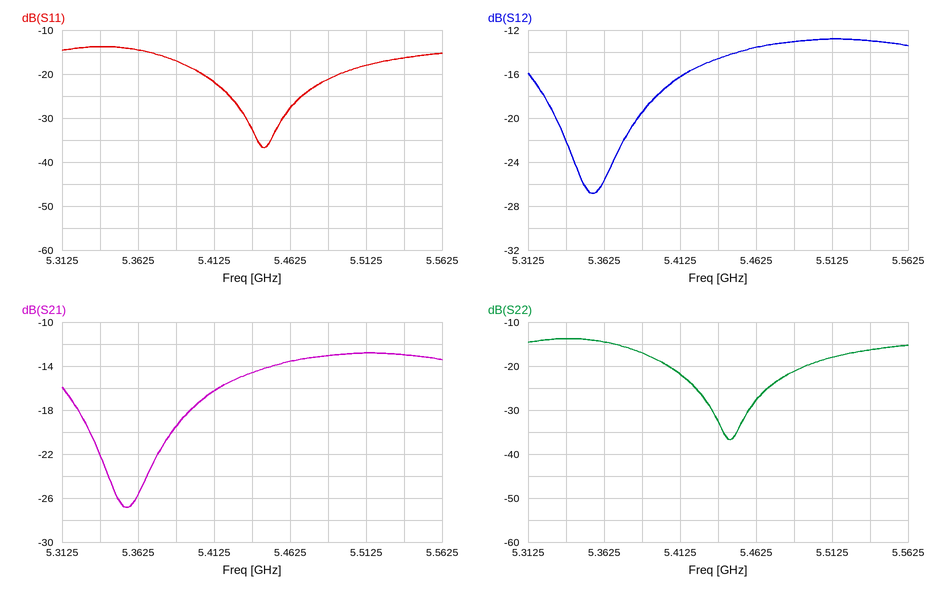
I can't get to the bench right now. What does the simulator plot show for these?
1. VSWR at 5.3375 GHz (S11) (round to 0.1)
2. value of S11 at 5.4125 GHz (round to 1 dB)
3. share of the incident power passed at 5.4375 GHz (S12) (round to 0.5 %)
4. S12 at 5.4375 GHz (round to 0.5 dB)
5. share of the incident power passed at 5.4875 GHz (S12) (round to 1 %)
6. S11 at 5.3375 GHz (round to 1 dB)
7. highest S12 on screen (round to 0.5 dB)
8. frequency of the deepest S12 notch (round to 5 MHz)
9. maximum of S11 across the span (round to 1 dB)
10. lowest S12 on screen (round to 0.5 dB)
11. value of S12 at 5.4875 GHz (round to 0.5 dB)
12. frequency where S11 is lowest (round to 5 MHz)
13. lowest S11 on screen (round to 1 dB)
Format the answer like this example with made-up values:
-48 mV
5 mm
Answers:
1.5
-22 dB
3.5 %
-14.5 dB
5 %
-14 dB
-13.0 dB
5.355 GHz
-14 dB
-27.0 dB
-13.0 dB
5.445 GHz
-37 dB
